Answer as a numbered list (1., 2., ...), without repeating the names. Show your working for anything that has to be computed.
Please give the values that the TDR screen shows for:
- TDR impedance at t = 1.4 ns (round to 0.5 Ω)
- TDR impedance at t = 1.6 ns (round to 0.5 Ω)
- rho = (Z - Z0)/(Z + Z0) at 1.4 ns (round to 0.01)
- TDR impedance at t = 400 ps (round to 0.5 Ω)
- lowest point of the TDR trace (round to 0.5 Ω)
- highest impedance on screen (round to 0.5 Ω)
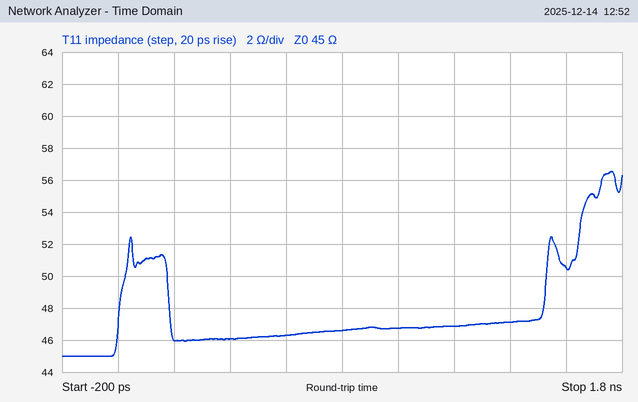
1. 47.0 Ω
2. 50.5 Ω
3. (47 − 45)/(47 + 45) ≈ +0.02
4. 46.0 Ω
5. 45.0 Ω
6. 56.5 Ω
